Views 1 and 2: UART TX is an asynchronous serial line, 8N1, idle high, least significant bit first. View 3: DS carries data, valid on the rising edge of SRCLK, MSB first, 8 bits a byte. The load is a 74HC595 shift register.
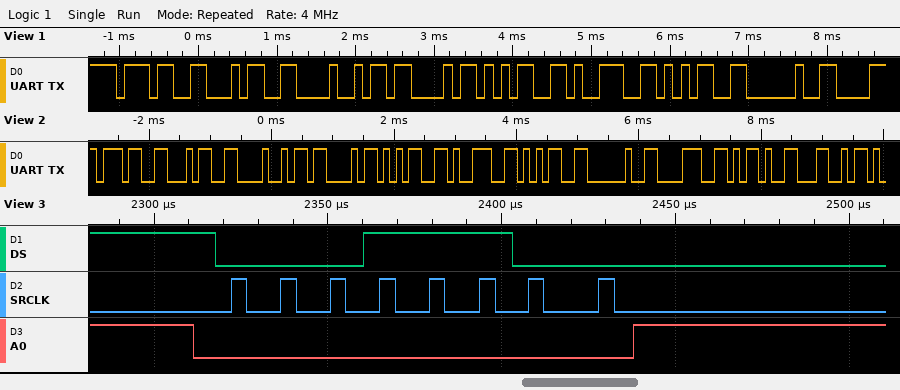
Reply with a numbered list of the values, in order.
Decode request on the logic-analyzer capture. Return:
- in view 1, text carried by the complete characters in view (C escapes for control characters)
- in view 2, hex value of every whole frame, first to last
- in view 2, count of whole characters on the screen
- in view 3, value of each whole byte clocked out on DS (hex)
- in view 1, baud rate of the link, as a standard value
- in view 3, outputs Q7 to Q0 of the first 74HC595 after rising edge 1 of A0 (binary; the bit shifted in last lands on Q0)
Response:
1. "74HC595 "
2. 0x37 0x34 0x48 0x43 0x35 0x39 0x35 0x20 0x38 0x2D 0x4C
3. 11
4. 0x1C
5. 9600 baud
6. 00011100
